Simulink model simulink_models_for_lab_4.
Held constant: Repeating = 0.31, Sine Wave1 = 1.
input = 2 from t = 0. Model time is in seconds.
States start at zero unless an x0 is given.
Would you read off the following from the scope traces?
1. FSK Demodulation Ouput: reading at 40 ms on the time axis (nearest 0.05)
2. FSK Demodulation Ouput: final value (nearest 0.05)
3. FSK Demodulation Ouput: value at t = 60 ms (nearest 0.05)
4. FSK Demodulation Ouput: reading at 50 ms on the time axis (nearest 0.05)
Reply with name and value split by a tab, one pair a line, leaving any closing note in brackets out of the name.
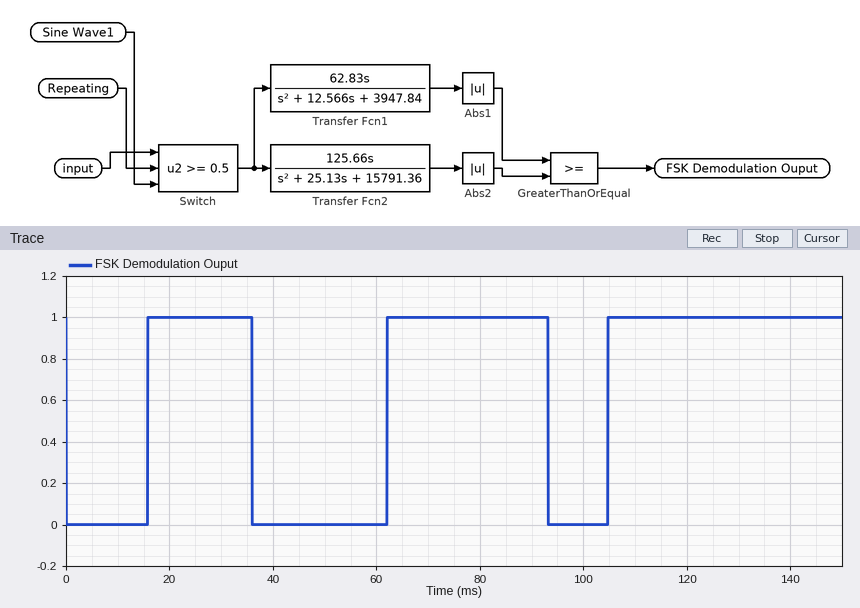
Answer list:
FSK Demodulation Ouput: reading at 40 ms on the time axis	0.00
FSK Demodulation Ouput: final value	1.00
FSK Demodulation Ouput: value at t = 60 ms	0.00
FSK Demodulation Ouput: reading at 50 ms on the time axis	0.00
